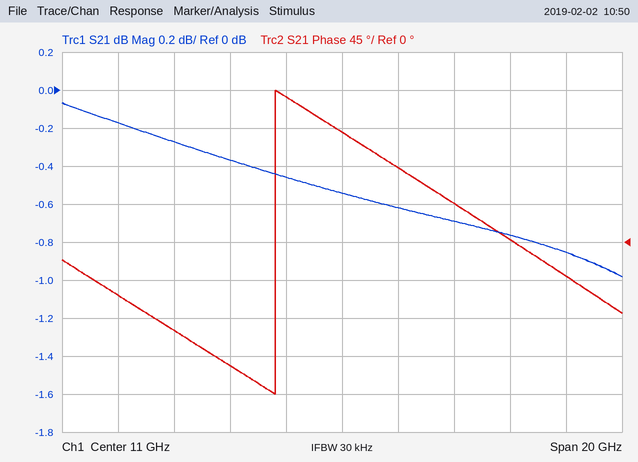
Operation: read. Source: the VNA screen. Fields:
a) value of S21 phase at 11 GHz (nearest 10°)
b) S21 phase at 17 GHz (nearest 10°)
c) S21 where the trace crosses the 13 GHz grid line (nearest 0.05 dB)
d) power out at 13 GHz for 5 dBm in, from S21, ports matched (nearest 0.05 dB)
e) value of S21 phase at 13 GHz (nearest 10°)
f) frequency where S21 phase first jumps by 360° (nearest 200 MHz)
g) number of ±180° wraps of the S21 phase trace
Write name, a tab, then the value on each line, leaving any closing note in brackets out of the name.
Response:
value of S21 phase at 11 GHz	130°
S21 phase at 17 GHz	0°
S21 where the trace crosses the 13 GHz grid line	-0.60 dB
power out at 13 GHz for 5 dBm in, from S21, ports matched	4.40 dBm
value of S21 phase at 13 GHz	90°
frequency where S21 phase first jumps by 360°	8.6 GHz
number of ±180° wraps of the S21 phase trace	1
